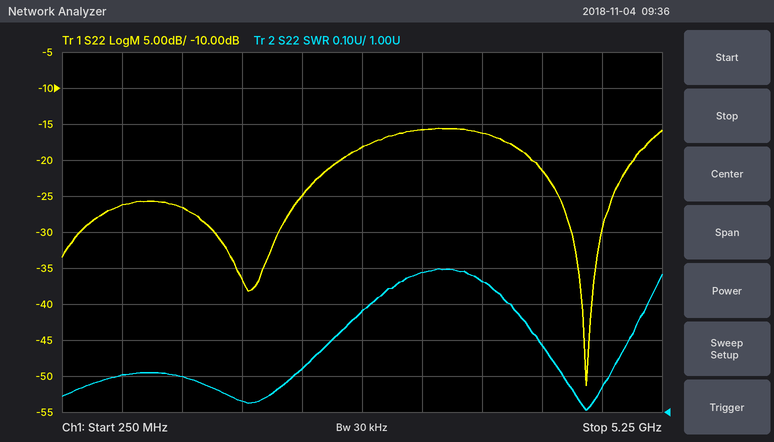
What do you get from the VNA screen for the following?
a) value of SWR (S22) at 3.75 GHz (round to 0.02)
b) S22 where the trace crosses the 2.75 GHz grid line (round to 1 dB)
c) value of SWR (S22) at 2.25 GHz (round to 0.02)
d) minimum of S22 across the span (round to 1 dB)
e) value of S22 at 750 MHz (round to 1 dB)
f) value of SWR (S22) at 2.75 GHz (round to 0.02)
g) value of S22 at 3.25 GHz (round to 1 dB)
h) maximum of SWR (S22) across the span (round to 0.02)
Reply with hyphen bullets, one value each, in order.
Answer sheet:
- 1.36
- -18 dB
- 1.12
- -51 dB
- -26 dB
- 1.28
- -16 dB
- 1.40
